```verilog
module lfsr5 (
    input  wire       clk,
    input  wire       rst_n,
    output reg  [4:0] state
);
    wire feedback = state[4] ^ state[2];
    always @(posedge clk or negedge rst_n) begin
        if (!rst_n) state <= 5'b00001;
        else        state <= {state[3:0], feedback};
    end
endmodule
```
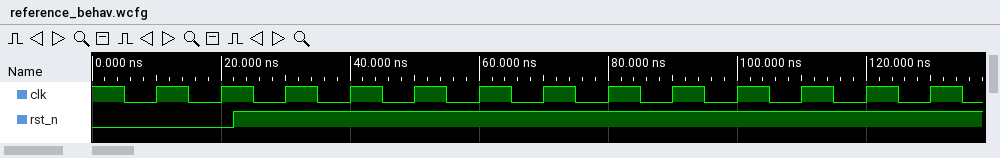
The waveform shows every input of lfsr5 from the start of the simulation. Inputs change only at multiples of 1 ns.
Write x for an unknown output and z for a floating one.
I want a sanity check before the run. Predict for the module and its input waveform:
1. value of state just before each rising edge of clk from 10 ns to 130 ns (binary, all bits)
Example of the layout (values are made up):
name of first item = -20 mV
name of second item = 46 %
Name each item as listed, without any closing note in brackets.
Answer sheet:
value of state just before each rising edge of clk from 10 ns to 130 ns = 00001, 00001, 00001, 00010, 00100, 01001, 10010, 00101, 01011, 10110, 01100, 11001, 10011
